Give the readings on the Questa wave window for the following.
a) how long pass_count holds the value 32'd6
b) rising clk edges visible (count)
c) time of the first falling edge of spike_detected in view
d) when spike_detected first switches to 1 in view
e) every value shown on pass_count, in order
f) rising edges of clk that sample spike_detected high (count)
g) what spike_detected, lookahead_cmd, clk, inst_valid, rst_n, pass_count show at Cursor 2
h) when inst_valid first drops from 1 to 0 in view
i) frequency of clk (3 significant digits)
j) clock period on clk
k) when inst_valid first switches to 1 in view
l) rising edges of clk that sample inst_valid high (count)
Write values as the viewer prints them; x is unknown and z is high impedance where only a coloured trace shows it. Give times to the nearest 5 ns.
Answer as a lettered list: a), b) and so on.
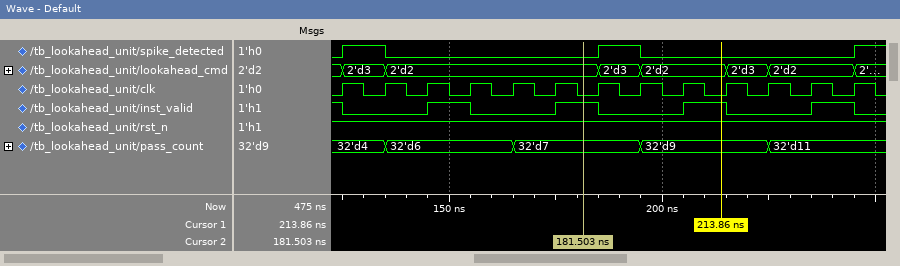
a) 30 ns
b) 13
c) 135 ns
d) 125 ns
e) 32'd4, 32'd6, 32'd7, 32'd9, 32'd11
f) 2
g) spike_detected=0, lookahead_cmd=2'd2, clk=0, inst_valid=1, rst_n=1, pass_count=32'd7
h) 125 ns
i) 100 MHz
j) 10 ns
k) 145 ns
l) 5
